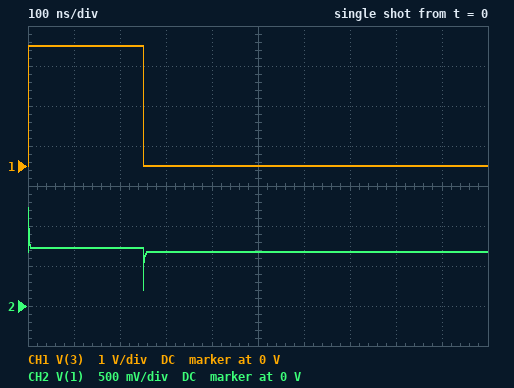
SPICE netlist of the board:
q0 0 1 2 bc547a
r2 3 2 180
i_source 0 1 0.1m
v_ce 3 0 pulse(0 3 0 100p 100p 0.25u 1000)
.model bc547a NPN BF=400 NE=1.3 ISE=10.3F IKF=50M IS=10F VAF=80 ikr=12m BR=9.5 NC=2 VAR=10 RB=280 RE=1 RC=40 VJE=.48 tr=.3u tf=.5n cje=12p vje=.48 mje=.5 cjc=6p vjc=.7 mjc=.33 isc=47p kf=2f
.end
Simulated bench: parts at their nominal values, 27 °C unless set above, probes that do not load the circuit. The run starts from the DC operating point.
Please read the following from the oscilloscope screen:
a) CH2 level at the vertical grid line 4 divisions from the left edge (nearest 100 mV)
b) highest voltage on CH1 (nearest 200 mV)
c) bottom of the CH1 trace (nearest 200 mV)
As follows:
700 mV
3.0 V
0 V
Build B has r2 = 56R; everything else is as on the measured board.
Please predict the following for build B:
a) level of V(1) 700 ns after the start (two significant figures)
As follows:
680 mV
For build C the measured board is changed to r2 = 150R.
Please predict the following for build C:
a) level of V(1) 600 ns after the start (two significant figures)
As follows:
680 mV
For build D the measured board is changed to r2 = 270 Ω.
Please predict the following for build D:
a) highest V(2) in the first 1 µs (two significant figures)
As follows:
2.7 V
